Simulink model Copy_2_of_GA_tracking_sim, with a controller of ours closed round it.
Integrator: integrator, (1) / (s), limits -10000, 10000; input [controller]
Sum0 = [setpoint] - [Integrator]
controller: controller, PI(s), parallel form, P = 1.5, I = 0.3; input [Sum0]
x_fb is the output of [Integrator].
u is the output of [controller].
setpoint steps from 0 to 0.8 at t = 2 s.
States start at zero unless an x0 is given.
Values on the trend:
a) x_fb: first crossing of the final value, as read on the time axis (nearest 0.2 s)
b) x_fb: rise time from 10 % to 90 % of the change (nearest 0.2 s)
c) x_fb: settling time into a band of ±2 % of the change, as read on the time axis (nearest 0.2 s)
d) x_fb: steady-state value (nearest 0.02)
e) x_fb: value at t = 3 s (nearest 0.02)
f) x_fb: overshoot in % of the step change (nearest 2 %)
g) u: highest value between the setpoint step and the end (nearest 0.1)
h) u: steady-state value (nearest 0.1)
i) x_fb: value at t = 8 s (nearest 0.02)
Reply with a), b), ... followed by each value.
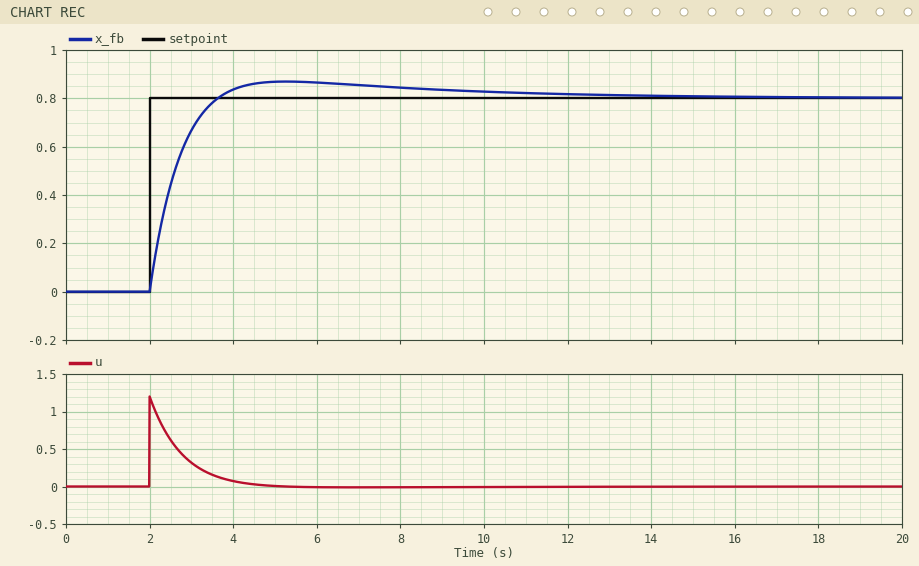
a) 3.6 s
b) 1.2 s
c) 12.4 s
d) 0.80
e) 0.66
f) 8 %
g) 1.2
h) 0.0
i) 0.84
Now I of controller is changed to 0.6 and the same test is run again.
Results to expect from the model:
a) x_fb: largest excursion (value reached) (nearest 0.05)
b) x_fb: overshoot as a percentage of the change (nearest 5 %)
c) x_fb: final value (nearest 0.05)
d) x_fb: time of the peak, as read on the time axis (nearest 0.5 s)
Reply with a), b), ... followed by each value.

a) 0.90
b) 15 %
c) 0.80
d) 4.5 s
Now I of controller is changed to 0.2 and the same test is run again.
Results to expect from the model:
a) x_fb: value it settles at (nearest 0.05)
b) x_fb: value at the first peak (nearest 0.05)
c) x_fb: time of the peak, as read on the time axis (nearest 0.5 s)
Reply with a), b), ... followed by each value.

a) 0.80
b) 0.85
c) 5.5 s
